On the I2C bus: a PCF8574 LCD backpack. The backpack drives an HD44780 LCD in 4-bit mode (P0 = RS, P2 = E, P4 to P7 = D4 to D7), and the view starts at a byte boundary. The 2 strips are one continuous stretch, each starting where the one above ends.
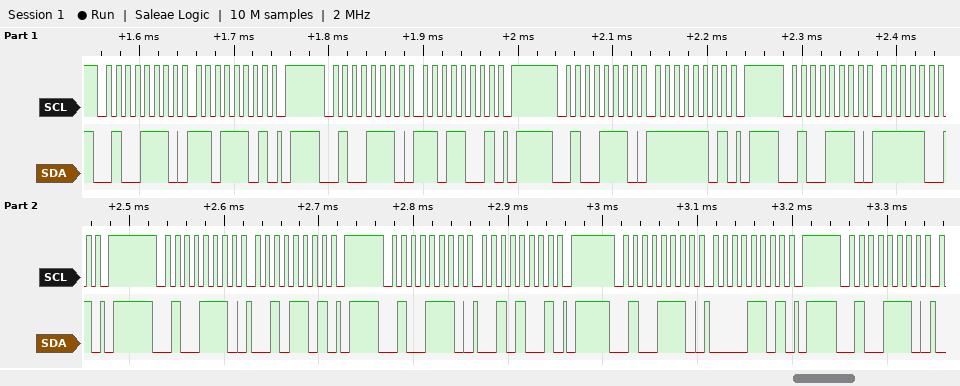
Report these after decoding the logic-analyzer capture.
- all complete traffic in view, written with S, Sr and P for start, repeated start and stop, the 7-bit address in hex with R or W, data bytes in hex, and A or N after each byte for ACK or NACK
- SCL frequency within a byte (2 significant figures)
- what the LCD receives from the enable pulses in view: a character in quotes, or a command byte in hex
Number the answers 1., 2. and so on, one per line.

1. S 27W A DD A P S 27W A D9 A P S 27W A FD A P S 27W A F9 A P S 27W A 2D A P S 27W A 29 A P S 27W A 0D A P S 27W A
2. 100 kHz
3. data 0xDF
